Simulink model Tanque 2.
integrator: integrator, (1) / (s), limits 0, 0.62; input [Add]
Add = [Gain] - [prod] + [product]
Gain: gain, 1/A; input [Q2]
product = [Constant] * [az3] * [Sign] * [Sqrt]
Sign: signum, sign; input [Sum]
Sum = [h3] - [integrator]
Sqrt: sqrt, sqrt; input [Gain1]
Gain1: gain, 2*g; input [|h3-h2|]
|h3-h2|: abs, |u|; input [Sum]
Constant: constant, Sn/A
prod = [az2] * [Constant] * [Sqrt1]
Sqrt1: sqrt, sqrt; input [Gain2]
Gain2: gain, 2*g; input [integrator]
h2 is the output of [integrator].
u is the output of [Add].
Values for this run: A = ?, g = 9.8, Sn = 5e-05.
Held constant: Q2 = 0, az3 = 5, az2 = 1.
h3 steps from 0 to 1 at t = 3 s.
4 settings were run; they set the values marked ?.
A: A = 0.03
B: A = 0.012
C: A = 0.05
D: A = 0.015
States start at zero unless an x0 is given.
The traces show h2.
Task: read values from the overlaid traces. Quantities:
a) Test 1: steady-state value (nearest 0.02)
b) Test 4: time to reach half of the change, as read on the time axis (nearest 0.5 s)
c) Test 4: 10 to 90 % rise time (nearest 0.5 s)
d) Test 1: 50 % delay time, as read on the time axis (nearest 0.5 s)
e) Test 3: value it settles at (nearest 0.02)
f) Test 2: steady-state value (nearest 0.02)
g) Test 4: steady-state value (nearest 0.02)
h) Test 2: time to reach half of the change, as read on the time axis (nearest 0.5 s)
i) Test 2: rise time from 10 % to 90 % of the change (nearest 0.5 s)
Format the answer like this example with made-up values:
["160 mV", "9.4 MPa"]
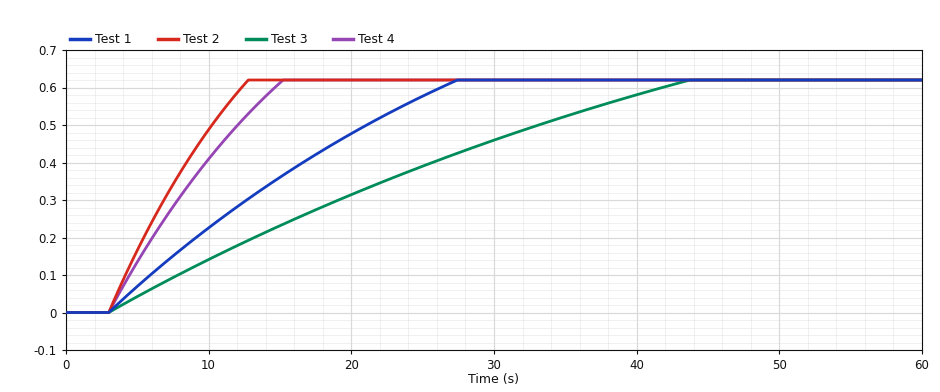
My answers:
["0.62", "8.0 s", "9.5 s", "13.0 s", "0.62", "0.62", "0.62", "7.0 s", "7.5 s"]
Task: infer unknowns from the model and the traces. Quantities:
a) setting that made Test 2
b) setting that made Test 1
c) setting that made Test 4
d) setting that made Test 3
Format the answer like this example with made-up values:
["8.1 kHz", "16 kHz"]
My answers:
["B", "A", "D", "C"]
